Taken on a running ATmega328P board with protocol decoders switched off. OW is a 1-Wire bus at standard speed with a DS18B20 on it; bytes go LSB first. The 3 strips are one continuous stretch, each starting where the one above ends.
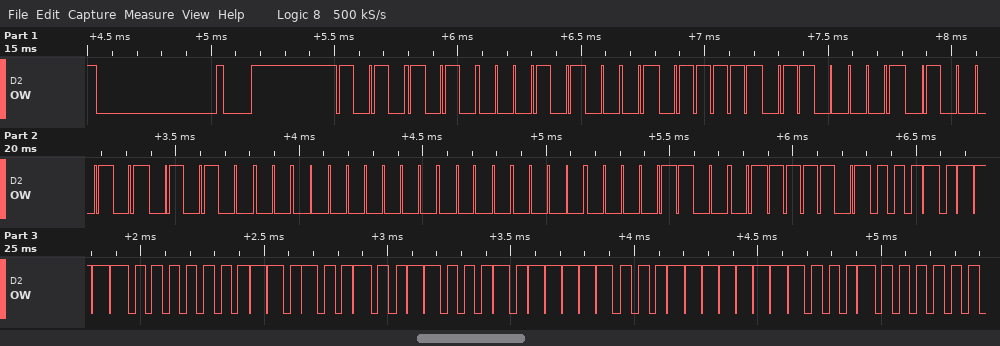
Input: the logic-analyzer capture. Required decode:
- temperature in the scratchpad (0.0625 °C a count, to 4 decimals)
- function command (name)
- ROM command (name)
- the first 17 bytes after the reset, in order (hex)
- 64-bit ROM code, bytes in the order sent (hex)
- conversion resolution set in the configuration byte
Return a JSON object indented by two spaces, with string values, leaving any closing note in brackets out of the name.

{
  "temperature in the scratchpad": "30.5000 °C",
  "function command": "Read Scratchpad",
  "ROM command": "Match ROM",
  "the first 17 bytes after the reset, in order": "55 28 FA 86 A2 0A 00 00 30 BE E8 01 4B 46 1F FF 08",
  "64-bit ROM code, bytes in the order sent": "28 FA 86 A2 0A 00 00 30",
  "conversion resolution set in the configuration byte": "9 bits"
}
